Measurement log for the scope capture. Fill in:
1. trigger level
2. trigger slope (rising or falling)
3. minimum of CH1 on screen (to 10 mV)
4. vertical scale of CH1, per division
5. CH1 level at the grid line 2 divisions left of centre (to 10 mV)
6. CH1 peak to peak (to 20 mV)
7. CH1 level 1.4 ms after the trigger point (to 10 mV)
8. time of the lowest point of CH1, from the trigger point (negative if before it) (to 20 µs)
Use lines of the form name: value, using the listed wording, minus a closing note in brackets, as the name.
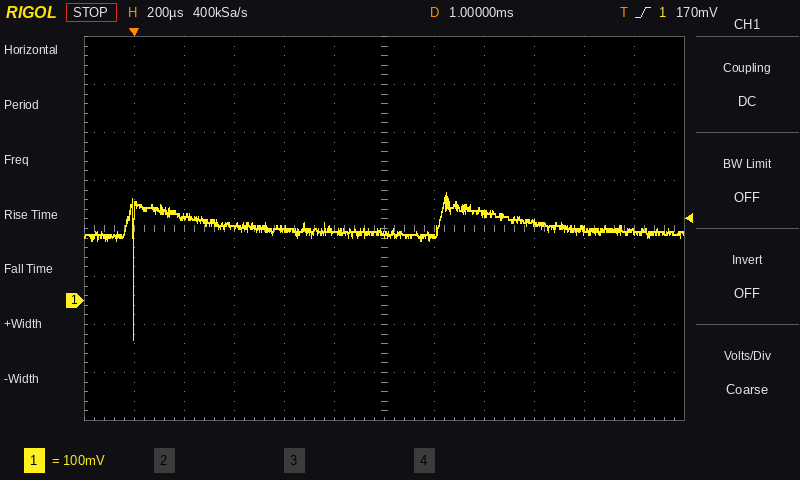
trigger level: 170 mV
trigger slope: rising
minimum of CH1 on screen: -80 mV
vertical scale of CH1, per division: 100 mV
CH1 level at the grid line 2 divisions left of centre: 150 mV
CH1 peak to peak: 300 mV
CH1 level 1.4 ms after the trigger point: 180 mV
time of the lowest point of CH1, from the trigger point (negative if before it): 0 µs
